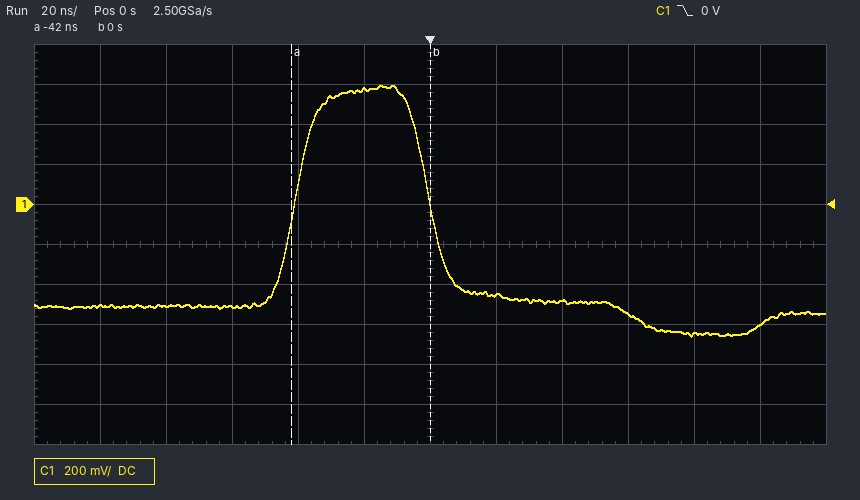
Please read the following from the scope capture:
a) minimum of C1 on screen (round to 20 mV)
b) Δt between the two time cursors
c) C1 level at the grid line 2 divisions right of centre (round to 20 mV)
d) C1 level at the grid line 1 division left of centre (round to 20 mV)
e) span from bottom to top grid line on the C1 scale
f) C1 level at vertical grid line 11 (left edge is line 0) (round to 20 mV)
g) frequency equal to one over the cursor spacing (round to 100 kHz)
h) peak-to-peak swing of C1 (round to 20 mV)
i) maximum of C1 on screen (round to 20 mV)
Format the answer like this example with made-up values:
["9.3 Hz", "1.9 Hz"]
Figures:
["-660 mV", "42 ns", "-480 mV", "580 mV", "2 V", "-600 mV", "23.8 MHz", "1.26 V", "600 mV"]
